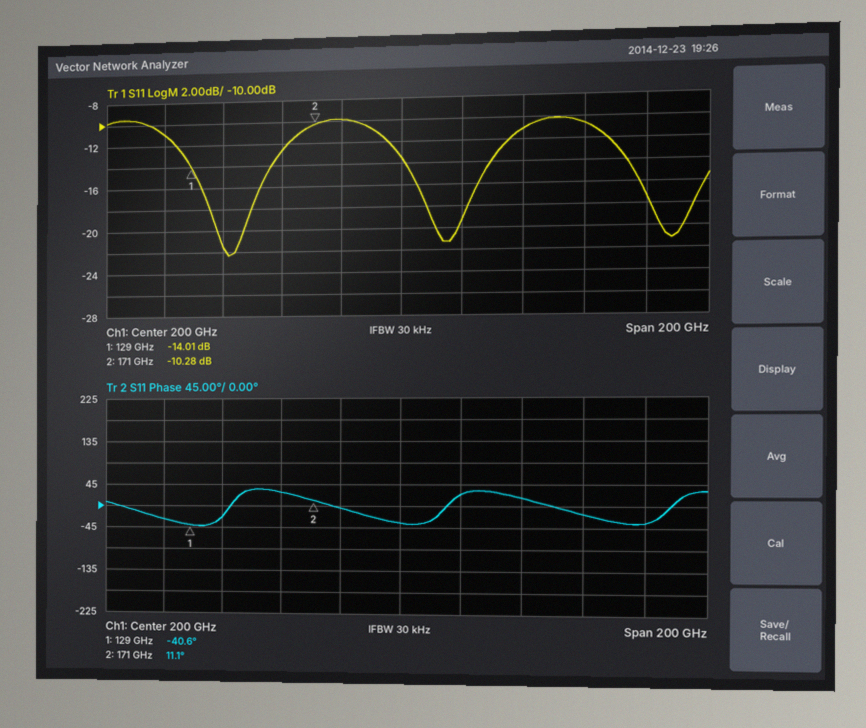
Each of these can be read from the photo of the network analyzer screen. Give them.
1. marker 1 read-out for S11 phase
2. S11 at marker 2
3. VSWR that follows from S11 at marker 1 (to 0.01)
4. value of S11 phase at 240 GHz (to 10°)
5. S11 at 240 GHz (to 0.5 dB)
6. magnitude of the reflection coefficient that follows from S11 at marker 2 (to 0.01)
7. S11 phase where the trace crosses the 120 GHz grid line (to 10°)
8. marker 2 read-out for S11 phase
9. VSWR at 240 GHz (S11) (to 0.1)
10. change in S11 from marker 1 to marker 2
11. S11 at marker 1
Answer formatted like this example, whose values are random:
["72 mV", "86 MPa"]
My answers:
["-40.6°", "-10.28 dB", "1.50", "20°", "-11.0 dB", "0.31", "-30°", "11.1°", "1.8", "3.73 dB", "-14.01 dB"]
